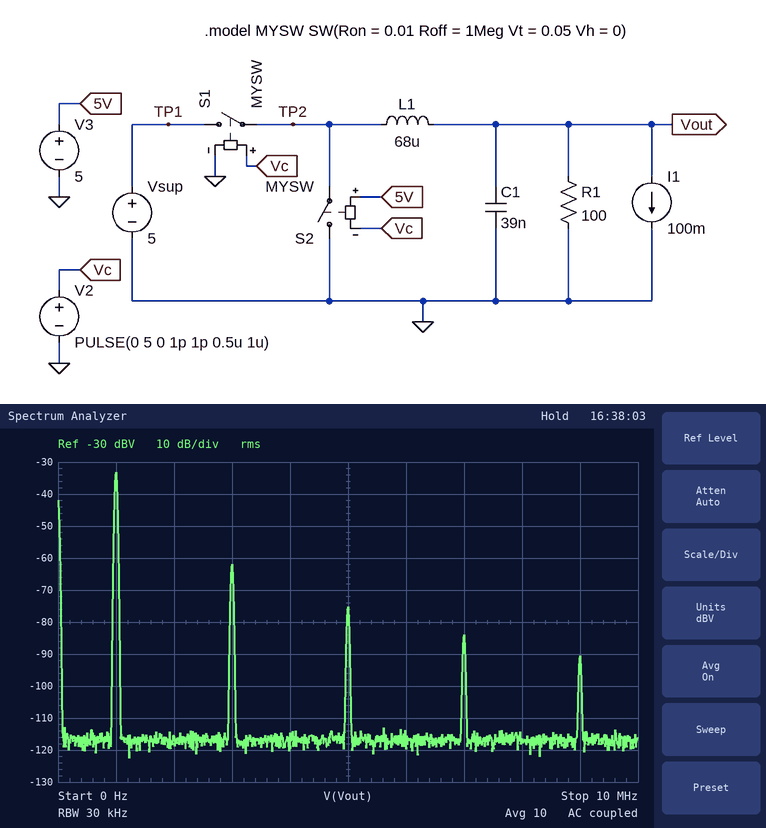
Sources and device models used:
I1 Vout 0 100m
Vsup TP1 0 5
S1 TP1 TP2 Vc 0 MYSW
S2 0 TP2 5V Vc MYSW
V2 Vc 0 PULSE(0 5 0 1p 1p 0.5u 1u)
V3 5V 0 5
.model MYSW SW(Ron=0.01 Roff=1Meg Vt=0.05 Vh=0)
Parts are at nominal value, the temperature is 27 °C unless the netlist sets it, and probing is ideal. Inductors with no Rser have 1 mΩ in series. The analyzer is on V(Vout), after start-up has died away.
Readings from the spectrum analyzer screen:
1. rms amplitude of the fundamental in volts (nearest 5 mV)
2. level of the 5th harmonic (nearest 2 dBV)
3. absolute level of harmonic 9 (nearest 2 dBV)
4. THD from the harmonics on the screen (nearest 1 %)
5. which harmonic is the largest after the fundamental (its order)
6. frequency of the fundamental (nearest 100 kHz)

20 mV
-76 dBV
-90 dBV
4 %
3
1.0 MHz
